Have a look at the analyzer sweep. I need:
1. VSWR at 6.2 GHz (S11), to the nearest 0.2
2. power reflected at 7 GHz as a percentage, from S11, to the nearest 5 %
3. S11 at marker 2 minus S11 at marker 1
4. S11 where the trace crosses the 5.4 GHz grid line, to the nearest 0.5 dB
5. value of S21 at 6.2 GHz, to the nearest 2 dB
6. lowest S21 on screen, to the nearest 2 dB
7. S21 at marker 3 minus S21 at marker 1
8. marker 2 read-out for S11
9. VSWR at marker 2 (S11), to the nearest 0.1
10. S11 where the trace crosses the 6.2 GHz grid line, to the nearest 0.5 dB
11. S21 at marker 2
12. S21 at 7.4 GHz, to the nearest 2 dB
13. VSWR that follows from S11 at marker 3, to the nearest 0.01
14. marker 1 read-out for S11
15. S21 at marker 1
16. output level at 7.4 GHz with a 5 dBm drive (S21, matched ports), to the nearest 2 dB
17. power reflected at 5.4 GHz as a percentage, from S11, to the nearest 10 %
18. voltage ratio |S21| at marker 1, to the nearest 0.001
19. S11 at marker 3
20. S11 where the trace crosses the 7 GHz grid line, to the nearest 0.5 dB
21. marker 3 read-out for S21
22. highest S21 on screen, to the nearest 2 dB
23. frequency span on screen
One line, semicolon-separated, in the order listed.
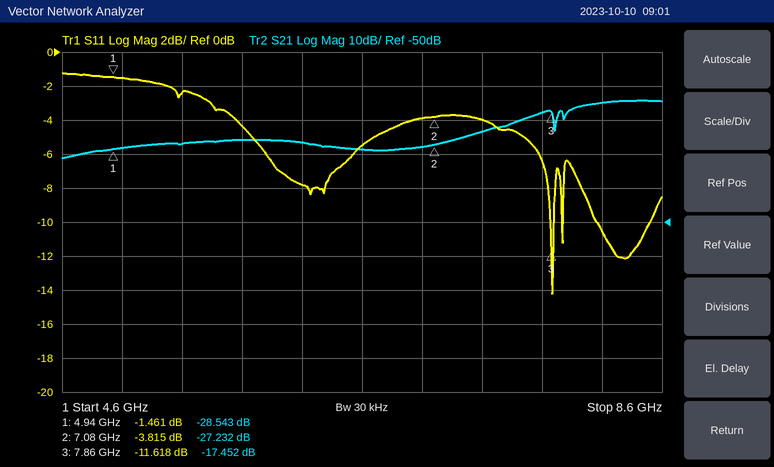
2.4; 40 %; -2.354 dB; -2.5 dB; -26 dB; -32 dB; 11.091 dB; -3.815 dB; 4.6; -8.0 dB; -27.232 dB; -24 dB; 1.71; -1.461 dB; -28.543 dB; -18 dBm; 60 %; 0.037; -11.618 dB; -4.0 dB; -17.452 dB; -14 dB; 4 GHz
